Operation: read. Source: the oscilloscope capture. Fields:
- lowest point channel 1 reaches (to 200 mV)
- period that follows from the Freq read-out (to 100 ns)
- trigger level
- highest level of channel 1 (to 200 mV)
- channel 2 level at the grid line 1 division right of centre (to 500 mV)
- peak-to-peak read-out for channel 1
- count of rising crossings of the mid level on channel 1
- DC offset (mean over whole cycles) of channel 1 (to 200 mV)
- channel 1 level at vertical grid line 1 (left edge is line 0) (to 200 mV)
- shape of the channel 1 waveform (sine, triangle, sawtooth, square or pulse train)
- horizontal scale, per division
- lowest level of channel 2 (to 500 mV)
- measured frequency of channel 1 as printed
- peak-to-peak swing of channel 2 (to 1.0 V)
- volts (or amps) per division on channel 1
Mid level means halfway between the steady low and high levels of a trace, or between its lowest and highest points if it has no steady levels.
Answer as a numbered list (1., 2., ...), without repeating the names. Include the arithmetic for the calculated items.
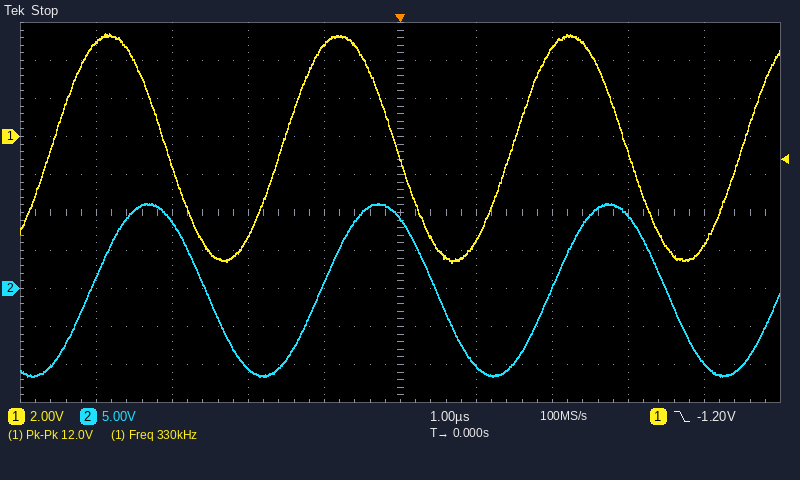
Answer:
1. -6.6 V
2. 1 / 330 kHz ≈ 3.0 µs
3. -1.20 V
4. 5.4 V
5. -10.0 V
6. 12.0 V
7. 4
8. (5.4 V + (-6.6 V)) / 2 ≈ -600 mV
9. 5.0 V
10. sine
11. 1 µs
12. -11.5 V
13. 330 kHz
14. 23.0 V
15. 2 V
